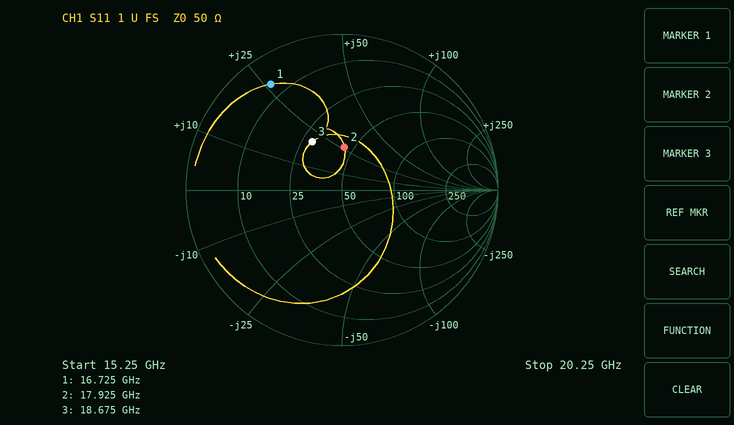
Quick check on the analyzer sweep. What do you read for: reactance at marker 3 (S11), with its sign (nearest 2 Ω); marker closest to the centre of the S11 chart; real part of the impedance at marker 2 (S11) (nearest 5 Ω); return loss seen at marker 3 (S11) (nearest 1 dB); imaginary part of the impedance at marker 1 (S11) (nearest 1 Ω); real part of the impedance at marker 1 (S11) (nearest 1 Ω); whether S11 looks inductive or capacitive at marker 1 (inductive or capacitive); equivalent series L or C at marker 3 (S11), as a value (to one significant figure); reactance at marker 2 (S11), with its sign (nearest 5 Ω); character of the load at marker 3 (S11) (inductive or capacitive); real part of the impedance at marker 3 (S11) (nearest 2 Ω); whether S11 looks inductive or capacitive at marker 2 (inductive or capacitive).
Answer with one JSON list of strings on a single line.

["+20 Ω", "marker 2", "45 Ω", "9 dB", "+26 Ω", "6 Ω", "inductive", "200 pH", "+25 Ω", "inductive", "28 Ω", "inductive"]
